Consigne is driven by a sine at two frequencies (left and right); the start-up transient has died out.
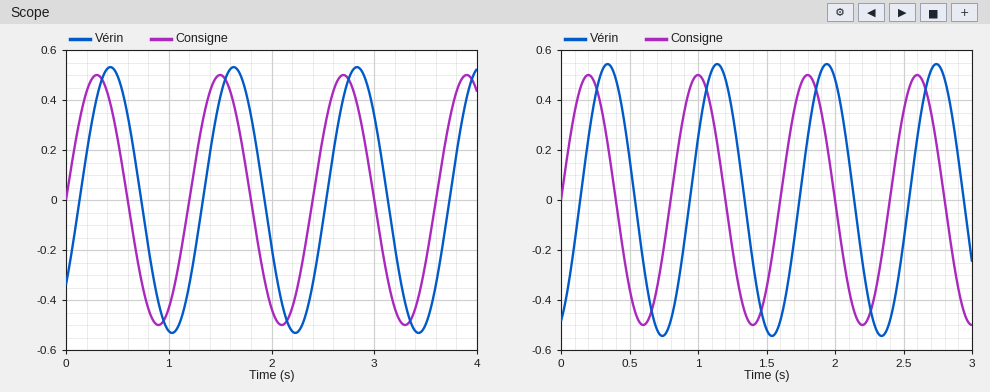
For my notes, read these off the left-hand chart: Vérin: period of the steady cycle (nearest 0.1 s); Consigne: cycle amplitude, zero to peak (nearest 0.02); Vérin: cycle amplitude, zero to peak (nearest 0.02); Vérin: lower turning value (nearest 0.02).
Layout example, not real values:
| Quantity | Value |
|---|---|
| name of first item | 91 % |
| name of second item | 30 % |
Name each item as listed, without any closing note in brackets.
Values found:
| Quantity | Value |
|---|---|
| Vérin: period of the steady cycle | 1.2 s |
| Consigne: cycle amplitude, zero to peak | 0.50 |
| Vérin: cycle amplitude, zero to peak | 0.54 |
| Vérin: lower turning value | -0.54 |
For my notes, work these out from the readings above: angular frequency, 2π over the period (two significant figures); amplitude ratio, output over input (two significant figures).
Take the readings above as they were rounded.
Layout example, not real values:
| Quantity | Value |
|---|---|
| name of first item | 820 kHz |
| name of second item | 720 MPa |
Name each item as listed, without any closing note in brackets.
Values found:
| Quantity | Value |
|---|---|
| angular frequency, 2π over the period | 5.2 rad/s |
| amplitude ratio, output over input | 1.1 |
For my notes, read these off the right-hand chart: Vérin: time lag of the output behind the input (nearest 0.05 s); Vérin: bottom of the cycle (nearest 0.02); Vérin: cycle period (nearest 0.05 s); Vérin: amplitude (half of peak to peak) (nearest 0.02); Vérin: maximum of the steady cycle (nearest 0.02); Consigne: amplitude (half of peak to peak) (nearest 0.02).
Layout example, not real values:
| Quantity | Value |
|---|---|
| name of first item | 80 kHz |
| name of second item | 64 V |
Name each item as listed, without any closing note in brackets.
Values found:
| Quantity | Value |
|---|---|
| Vérin: time lag of the output behind the input | 0.15 s |
| Vérin: bottom of the cycle | -0.54 |
| Vérin: cycle period | 0.80 s |
| Vérin: amplitude (half of peak to peak) | 0.54 |
| Vérin: maximum of the steady cycle | 0.54 |
| Consigne: amplitude (half of peak to peak) | 0.50 |
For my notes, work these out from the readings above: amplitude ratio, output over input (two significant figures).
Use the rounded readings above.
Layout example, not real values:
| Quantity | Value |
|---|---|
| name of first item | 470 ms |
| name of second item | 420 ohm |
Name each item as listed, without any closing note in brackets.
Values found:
| Quantity | Value |
|---|---|
| amplitude ratio, output over input | 1.1 |
